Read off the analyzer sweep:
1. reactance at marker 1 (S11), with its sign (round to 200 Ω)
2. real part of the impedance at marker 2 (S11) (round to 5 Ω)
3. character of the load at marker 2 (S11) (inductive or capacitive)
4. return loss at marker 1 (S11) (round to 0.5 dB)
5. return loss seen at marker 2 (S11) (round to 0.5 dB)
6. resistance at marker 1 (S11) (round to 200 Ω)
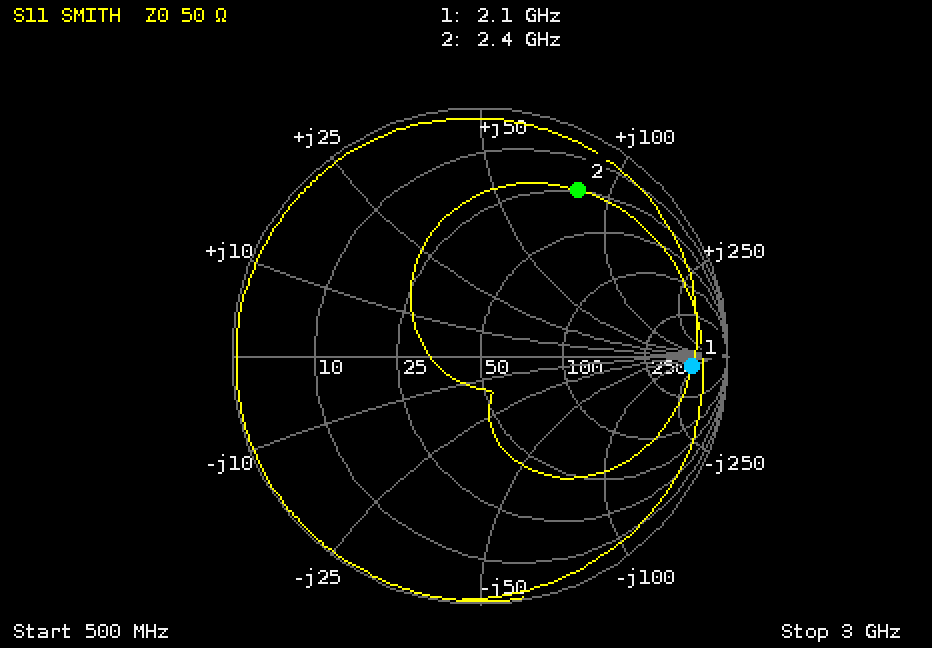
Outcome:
-200 Ω
25 Ω
inductive
1.5 dB
2.0 dB
600 Ω
